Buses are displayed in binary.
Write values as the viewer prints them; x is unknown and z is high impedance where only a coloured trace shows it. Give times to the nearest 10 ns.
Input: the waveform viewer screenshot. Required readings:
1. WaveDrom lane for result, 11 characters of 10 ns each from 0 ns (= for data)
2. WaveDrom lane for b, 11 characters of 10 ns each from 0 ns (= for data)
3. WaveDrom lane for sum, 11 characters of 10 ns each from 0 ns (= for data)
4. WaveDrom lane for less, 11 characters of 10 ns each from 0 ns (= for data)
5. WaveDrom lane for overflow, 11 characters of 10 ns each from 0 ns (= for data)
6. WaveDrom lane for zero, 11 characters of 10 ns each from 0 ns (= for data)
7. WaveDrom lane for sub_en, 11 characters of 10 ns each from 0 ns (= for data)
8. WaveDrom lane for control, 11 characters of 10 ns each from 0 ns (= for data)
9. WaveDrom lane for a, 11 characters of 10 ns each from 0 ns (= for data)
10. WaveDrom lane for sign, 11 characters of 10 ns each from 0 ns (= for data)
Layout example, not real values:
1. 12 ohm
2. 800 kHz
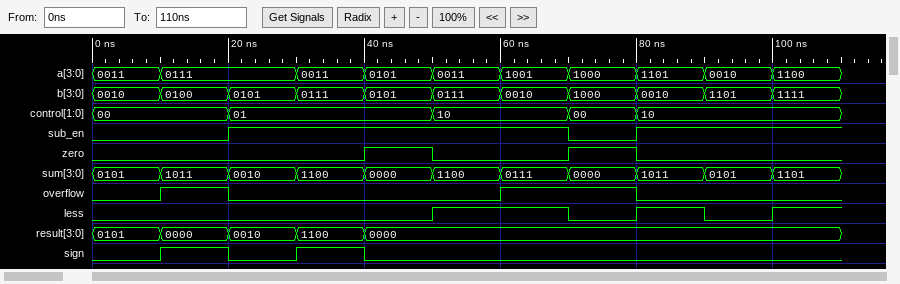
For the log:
1. {name: 'result', wave: '=====......', data: '0101 0000 0010 1100 0000'}
2. {name: 'b', wave: '===========', data: '0010 0100 0101 0111 0101 0111 0010 1000 0010 1101 1111'}
3. {name: 'sum', wave: '===========', data: '0101 1011 0010 1100 0000 1100 0111 0000 1011 0101 1101'}
4. {name: 'less', wave: '0....1.0101'}
5. {name: 'overflow', wave: '010...1.0..'}
6. {name: 'zero', wave: '0...10.10..'}
7. {name: 'sub_en', wave: '0.1....01..'}
8. {name: 'control', wave: '=.=..=.==..', data: '00 01 10 00 10'}
9. {name: 'a', wave: '==.========', data: '0011 0111 0011 0101 0011 1001 1000 1101 0010 1100'}
10. {name: 'sign', wave: '01010......'}
